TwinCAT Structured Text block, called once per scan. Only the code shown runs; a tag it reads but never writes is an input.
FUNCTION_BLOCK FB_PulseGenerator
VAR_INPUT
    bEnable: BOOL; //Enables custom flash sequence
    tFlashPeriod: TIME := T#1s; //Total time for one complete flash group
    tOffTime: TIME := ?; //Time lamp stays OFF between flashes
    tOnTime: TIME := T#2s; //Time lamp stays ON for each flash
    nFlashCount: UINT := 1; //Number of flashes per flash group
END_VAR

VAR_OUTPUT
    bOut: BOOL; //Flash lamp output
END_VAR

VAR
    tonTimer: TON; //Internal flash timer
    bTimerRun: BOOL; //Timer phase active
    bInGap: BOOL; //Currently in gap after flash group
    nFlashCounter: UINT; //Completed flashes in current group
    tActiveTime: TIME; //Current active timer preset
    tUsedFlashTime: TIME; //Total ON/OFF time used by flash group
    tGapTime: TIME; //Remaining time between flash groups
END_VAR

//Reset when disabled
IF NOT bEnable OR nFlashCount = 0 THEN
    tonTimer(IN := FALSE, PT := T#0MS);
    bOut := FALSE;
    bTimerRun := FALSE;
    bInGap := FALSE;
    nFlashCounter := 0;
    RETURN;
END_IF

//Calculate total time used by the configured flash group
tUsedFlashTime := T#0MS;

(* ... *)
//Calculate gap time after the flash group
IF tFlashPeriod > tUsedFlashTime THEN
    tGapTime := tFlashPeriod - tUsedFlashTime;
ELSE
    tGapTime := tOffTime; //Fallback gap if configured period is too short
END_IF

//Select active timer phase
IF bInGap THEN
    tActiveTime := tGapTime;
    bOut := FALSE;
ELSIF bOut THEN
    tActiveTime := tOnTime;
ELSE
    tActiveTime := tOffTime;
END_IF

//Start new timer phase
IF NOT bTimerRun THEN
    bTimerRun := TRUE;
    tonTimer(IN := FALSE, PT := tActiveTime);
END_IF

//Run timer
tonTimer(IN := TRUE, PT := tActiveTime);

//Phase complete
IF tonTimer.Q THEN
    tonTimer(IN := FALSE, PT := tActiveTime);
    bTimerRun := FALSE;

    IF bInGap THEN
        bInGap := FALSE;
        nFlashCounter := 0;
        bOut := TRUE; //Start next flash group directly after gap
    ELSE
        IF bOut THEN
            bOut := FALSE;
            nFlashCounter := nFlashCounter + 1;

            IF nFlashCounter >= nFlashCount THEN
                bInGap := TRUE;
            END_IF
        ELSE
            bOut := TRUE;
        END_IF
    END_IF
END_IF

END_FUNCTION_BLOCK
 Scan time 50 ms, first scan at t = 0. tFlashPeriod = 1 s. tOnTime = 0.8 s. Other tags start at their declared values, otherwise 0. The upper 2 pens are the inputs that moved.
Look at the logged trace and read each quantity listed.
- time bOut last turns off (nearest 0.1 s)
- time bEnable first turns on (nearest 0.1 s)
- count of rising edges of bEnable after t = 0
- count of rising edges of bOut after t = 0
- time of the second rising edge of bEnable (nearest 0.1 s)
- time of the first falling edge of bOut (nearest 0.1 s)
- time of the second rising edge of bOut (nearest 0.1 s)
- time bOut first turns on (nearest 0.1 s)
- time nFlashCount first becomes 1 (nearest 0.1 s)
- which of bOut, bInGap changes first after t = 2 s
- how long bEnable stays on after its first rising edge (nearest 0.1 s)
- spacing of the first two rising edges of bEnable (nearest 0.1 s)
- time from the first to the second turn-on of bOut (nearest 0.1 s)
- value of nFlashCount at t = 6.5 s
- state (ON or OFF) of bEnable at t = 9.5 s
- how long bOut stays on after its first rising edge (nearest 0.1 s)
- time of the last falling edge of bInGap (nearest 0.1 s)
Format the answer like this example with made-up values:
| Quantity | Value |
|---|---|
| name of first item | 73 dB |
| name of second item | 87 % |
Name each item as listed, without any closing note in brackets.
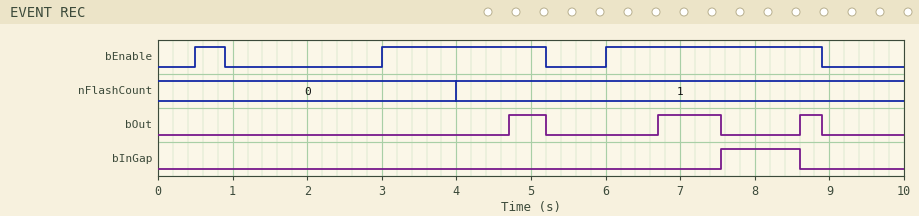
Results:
| Quantity | Value |
|---|---|
| time bOut last turns off | 8.9 s |
| time bEnable first turns on | 0.5 s |
| count of rising edges of bEnable after t = 0 | 3 |
| count of rising edges of bOut after t = 0 | 3 |
| time of the second rising edge of bEnable | 3.0 s |
| time of the first falling edge of bOut | 5.2 s |
| time of the second rising edge of bOut | 6.7 s |
| time bOut first turns on | 4.7 s |
| time nFlashCount first becomes 1 | 4.0 s |
| which of bOut, bInGap changes first after t = 2 s | bOut |
| how long bEnable stays on after its first rising edge | 0.4 s |
| spacing of the first two rising edges of bEnable | 2.5 s |
| time from the first to the second turn-on of bOut | 2.0 s |
| value of nFlashCount at t = 6.5 s | 1 |
| state (ON or OFF) of bEnable at t = 9.5 s | OFF |
| how long bOut stays on after its first rising edge | 0.5 s |
| time of the last falling edge of bInGap | 8.6 s |
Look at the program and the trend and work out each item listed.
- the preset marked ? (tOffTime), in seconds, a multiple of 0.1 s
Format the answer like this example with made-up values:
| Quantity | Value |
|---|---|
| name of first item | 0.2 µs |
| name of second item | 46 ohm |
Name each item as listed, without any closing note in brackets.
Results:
| Quantity | Value |
|---|---|
| the preset marked ? (tOffTime), in seconds, a multiple of 0.1 s | 0.7 s |
